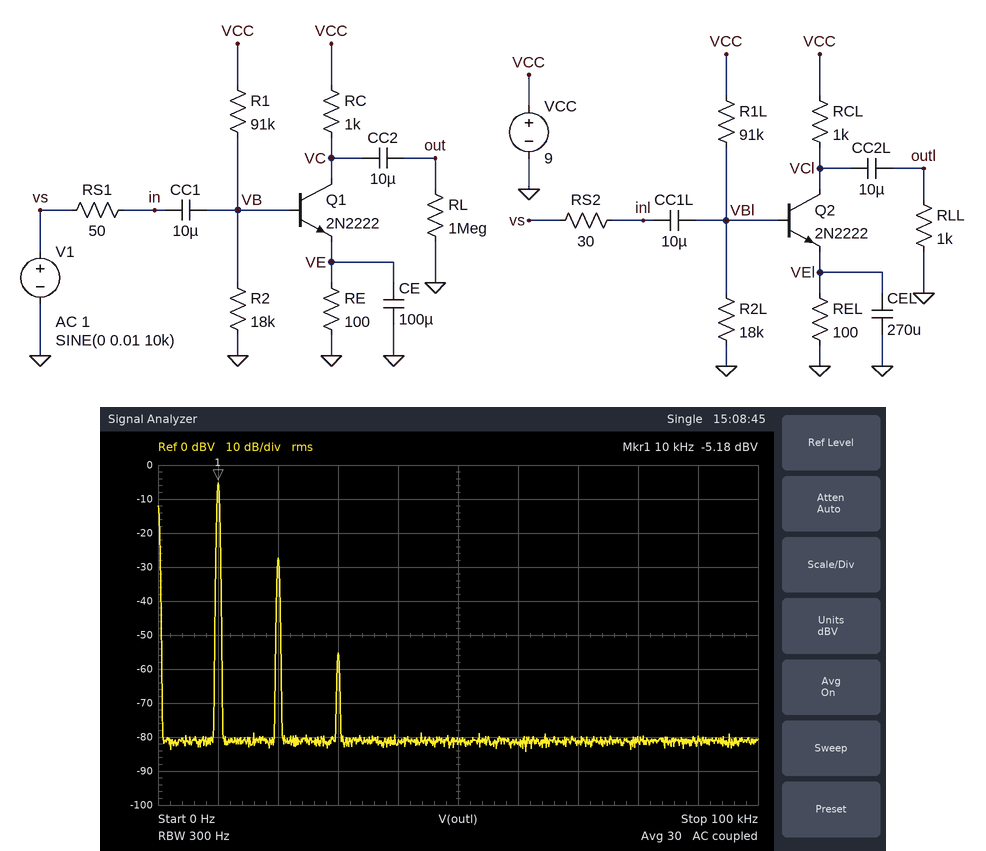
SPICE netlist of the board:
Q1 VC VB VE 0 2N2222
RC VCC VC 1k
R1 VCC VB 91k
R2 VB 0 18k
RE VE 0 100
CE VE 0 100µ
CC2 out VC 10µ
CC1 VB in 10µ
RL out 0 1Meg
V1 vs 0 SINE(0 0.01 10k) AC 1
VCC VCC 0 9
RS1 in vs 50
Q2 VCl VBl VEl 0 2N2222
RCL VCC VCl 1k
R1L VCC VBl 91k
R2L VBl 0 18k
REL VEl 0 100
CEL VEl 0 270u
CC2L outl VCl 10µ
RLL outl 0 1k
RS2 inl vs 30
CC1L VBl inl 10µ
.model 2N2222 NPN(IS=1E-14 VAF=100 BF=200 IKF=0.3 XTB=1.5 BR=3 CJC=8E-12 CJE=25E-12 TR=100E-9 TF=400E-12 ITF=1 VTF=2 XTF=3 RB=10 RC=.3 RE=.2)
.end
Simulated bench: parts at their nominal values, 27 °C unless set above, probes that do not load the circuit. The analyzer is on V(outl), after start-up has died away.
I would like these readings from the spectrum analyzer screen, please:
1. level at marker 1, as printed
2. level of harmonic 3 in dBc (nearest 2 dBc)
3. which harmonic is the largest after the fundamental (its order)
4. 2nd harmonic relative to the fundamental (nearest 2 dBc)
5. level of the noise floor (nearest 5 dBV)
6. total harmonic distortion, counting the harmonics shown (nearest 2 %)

-5.18 dBV
-50 dBc
2
-22 dBc
-80 dBV
8 %
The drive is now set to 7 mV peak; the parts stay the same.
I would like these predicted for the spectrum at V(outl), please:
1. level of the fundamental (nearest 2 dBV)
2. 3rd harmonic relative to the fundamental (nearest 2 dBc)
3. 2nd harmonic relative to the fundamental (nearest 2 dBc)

-8 dBV
-56 dBc
-26 dBc
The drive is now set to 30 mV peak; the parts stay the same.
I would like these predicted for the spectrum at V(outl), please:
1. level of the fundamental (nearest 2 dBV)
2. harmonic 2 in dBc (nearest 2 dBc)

4 dBV
-12 dBc
